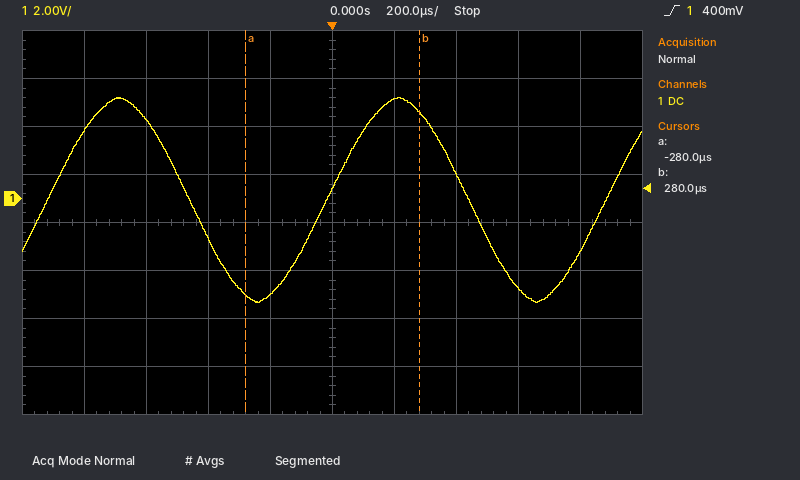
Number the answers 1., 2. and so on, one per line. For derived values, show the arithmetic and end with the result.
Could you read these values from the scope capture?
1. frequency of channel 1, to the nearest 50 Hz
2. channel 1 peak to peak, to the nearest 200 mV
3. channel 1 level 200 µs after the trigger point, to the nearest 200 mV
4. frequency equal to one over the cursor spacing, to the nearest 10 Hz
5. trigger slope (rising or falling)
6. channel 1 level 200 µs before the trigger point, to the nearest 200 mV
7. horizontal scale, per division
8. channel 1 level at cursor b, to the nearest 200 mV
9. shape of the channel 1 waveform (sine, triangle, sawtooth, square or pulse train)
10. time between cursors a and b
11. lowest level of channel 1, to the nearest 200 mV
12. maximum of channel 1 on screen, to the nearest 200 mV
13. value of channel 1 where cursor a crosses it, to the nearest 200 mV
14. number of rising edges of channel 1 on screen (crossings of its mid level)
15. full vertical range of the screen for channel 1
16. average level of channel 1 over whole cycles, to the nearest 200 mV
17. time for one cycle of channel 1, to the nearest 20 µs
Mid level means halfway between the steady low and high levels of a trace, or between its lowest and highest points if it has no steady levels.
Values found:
1. 1 / 900 µs ≈ 1.11 kHz, so 1.10 kHz to the nearest 50 Hz
2. 4.2 V − (-4.4 V) = 8.6 V
3. 4.2 V
4. 1 / 560 µs ≈ 1.79 kHz
5. rising
6. -4.0 V
7. 200 µs
8. 3.6 V
9. sine
10. 280 µs − (-280 µs) = 560 µs
11. -4.4 V
12. 4.2 V
13. -4.0 V
14. 3
15. 16 V
16. (4.2 V + (-4.4 V)) / 2 ≈ 0.0 V
17. 900 µs
